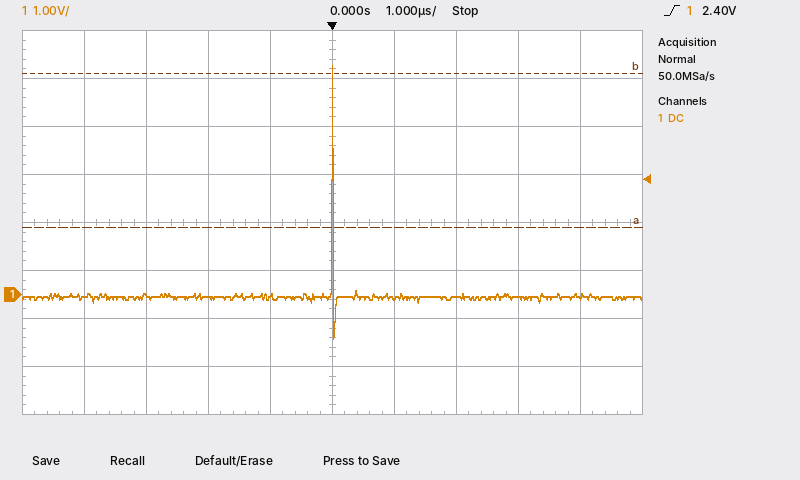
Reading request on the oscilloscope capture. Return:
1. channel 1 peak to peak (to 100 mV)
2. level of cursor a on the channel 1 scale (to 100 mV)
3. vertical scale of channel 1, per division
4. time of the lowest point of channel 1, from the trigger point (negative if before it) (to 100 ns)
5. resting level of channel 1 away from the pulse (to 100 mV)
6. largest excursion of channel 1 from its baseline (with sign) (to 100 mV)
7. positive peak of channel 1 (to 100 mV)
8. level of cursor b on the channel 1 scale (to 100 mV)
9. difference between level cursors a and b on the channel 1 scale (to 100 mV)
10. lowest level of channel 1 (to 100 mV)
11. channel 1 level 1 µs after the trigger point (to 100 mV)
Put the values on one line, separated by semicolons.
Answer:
5.7 V; 1.4 V; 1 V; 0.0 µs; 0.0 V; +4.8 V; 4.8 V; 4.6 V; 3.2 V; -900 mV; -100 mV
